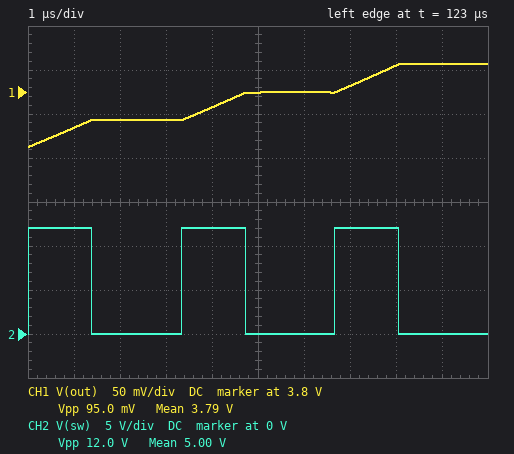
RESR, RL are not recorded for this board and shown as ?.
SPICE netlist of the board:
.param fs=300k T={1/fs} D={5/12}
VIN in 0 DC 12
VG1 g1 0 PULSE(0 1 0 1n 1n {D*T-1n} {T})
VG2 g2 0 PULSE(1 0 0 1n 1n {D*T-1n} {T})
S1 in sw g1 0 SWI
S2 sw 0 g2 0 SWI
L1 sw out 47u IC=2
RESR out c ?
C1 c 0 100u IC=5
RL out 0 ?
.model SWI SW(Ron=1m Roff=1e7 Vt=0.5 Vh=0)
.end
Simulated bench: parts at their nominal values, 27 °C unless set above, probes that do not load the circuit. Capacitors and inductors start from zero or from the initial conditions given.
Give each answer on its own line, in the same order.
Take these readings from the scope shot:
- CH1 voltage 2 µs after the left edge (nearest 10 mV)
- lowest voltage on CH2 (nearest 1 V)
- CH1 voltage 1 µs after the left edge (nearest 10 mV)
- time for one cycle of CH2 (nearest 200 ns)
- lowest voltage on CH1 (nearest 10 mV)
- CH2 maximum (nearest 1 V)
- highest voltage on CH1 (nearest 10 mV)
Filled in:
3.77 V
0 V
3.76 V
3.4 µs
3.74 V
12 V
3.83 V
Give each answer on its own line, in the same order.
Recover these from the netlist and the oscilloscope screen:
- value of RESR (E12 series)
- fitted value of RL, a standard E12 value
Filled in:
0.1 Ω
0.82 Ω
